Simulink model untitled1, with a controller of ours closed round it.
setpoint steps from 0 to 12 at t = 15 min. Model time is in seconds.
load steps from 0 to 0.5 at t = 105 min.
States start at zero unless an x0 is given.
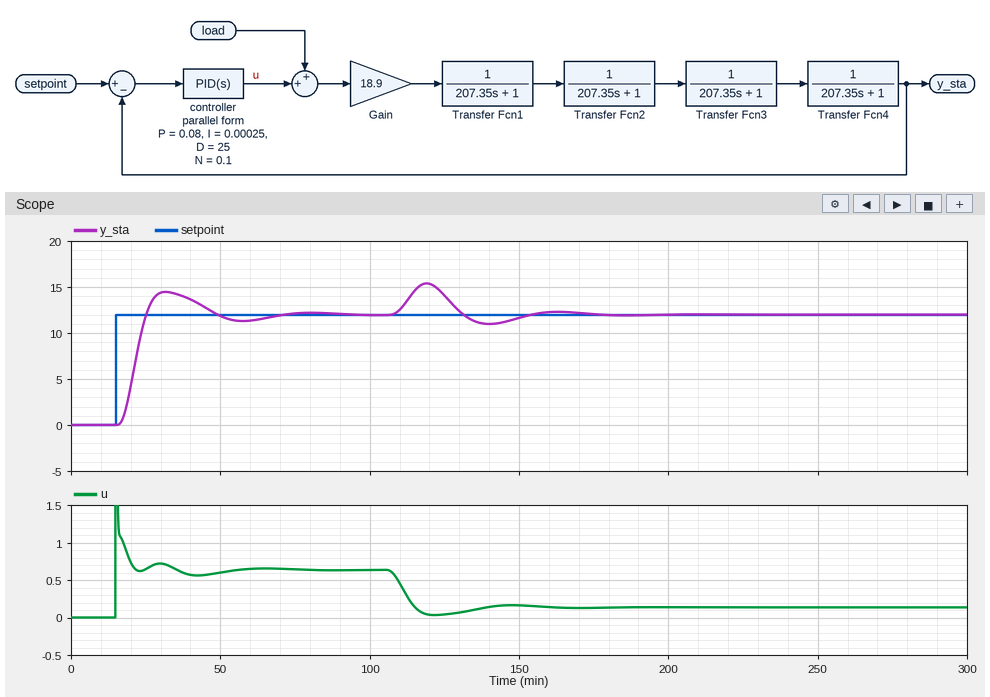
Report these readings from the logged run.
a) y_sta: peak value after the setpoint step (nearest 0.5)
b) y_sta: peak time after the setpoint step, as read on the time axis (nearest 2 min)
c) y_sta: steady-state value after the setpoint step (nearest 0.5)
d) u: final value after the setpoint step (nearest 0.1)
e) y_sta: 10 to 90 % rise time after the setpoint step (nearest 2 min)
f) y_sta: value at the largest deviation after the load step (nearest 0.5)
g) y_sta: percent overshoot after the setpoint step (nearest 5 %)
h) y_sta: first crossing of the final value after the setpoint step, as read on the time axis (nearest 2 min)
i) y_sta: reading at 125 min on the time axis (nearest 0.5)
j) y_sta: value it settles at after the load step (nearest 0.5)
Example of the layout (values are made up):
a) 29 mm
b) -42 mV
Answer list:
a) 14.5
b) 32 min
c) 12.0
d) 0.6
e) 6 min
f) 15.5
g) 20 %
h) 26 min
i) 14.0
j) 12.0
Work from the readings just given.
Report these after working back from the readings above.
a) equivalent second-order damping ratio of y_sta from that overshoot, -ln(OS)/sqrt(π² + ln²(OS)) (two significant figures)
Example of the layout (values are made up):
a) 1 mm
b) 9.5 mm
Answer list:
a) 0.46
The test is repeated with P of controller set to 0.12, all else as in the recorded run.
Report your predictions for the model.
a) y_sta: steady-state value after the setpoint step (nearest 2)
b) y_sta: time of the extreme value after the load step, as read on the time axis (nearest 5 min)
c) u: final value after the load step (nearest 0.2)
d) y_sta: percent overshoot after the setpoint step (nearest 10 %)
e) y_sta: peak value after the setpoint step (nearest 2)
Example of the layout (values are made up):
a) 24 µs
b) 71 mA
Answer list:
a) 12
b) 120 min
c) 0.2
d) 30 %
e) 16
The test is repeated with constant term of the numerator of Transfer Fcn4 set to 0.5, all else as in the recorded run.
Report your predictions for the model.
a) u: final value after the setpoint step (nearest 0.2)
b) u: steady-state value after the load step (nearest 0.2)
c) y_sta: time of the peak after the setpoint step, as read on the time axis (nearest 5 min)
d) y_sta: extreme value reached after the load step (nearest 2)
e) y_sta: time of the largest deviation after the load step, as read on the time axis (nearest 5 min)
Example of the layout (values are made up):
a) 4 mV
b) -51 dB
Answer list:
a) 1.2
b) 0.8
c) 45 min
d) 14
e) 120 min
